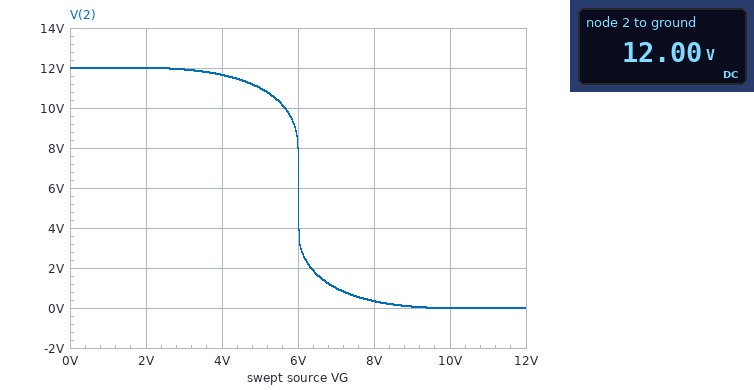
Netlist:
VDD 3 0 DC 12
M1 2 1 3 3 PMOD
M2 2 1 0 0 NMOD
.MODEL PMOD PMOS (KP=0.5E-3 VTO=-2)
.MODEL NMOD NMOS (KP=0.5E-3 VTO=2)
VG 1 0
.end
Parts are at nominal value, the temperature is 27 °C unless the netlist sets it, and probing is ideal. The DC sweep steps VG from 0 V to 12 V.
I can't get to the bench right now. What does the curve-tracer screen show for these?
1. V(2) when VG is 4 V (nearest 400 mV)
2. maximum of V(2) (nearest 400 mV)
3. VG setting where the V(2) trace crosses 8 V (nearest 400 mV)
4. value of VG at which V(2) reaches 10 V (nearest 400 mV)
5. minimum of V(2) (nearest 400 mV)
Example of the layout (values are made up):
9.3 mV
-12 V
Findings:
11.6 V
12.0 V
6.0 V
5.6 V
0 V
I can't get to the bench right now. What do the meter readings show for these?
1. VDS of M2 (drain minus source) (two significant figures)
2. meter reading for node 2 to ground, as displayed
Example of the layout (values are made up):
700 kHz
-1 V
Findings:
12 V
12.00 V
